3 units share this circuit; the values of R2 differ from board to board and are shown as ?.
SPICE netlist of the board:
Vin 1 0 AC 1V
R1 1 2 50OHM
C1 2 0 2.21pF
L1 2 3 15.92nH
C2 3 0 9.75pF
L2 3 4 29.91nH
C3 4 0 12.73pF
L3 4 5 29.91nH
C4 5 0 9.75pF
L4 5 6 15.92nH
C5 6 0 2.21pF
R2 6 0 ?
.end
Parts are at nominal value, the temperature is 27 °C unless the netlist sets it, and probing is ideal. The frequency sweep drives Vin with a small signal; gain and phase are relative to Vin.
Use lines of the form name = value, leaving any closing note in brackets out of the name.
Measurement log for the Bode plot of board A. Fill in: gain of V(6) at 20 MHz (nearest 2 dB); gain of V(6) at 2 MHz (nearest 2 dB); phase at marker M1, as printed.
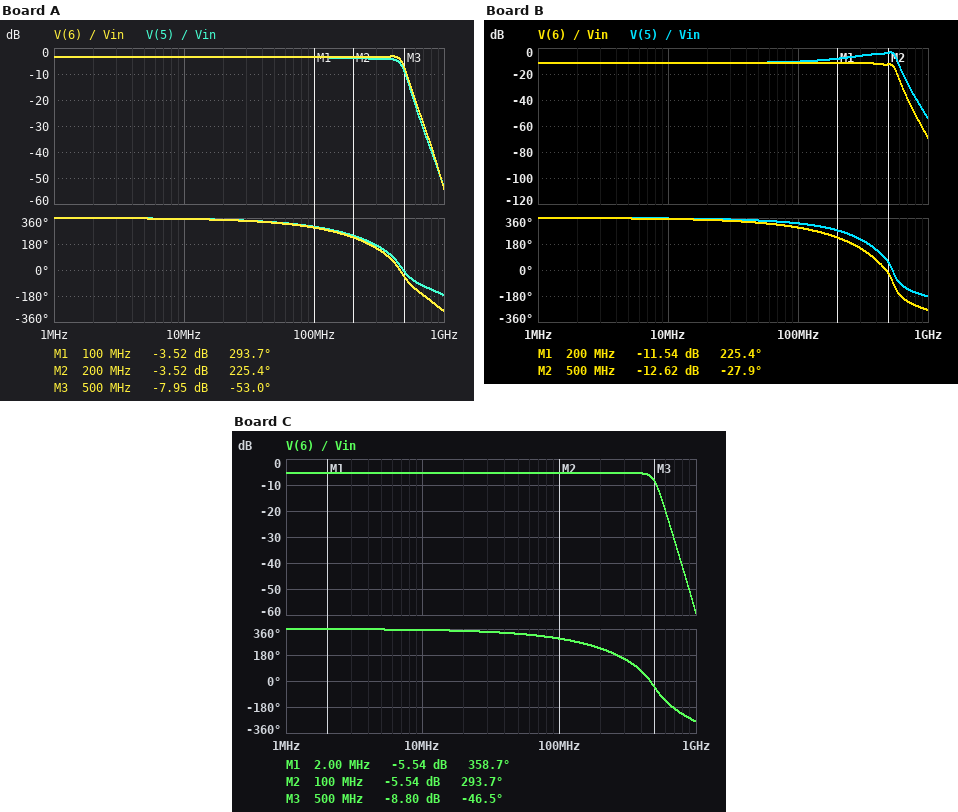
gain of V(6) at 20 MHz = -4 dB
gain of V(6) at 2 MHz = -4 dB
phase at marker M1, as printed = 293.7 deg
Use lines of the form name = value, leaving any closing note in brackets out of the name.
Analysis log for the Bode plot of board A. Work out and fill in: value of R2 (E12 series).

value of R2 = 100 Ω
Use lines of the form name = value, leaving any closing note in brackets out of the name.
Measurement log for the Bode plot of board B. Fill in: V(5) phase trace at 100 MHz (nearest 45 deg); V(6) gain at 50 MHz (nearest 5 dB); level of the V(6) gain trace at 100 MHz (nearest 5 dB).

V(5) phase trace at 100 MHz = 315 deg
V(6) gain at 50 MHz = -10 dB
level of the V(6) gain trace at 100 MHz = -10 dB
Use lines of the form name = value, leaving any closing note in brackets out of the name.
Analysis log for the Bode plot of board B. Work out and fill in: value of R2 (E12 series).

value of R2 = 18 Ω
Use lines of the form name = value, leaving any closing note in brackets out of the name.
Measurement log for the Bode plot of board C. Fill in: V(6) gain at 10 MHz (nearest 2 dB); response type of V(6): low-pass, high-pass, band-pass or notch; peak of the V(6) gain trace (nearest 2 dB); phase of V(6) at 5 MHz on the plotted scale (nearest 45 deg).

V(6) gain at 10 MHz = -6 dB
response type of V(6): low-pass, high-pass, band-pass or notch = low-pass
peak of the V(6) gain trace = -6 dB
phase of V(6) at 5 MHz on the plotted scale = 360 deg
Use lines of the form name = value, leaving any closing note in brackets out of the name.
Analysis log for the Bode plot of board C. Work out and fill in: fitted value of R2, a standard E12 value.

fitted value of R2, a standard E12 value = 56 Ω
